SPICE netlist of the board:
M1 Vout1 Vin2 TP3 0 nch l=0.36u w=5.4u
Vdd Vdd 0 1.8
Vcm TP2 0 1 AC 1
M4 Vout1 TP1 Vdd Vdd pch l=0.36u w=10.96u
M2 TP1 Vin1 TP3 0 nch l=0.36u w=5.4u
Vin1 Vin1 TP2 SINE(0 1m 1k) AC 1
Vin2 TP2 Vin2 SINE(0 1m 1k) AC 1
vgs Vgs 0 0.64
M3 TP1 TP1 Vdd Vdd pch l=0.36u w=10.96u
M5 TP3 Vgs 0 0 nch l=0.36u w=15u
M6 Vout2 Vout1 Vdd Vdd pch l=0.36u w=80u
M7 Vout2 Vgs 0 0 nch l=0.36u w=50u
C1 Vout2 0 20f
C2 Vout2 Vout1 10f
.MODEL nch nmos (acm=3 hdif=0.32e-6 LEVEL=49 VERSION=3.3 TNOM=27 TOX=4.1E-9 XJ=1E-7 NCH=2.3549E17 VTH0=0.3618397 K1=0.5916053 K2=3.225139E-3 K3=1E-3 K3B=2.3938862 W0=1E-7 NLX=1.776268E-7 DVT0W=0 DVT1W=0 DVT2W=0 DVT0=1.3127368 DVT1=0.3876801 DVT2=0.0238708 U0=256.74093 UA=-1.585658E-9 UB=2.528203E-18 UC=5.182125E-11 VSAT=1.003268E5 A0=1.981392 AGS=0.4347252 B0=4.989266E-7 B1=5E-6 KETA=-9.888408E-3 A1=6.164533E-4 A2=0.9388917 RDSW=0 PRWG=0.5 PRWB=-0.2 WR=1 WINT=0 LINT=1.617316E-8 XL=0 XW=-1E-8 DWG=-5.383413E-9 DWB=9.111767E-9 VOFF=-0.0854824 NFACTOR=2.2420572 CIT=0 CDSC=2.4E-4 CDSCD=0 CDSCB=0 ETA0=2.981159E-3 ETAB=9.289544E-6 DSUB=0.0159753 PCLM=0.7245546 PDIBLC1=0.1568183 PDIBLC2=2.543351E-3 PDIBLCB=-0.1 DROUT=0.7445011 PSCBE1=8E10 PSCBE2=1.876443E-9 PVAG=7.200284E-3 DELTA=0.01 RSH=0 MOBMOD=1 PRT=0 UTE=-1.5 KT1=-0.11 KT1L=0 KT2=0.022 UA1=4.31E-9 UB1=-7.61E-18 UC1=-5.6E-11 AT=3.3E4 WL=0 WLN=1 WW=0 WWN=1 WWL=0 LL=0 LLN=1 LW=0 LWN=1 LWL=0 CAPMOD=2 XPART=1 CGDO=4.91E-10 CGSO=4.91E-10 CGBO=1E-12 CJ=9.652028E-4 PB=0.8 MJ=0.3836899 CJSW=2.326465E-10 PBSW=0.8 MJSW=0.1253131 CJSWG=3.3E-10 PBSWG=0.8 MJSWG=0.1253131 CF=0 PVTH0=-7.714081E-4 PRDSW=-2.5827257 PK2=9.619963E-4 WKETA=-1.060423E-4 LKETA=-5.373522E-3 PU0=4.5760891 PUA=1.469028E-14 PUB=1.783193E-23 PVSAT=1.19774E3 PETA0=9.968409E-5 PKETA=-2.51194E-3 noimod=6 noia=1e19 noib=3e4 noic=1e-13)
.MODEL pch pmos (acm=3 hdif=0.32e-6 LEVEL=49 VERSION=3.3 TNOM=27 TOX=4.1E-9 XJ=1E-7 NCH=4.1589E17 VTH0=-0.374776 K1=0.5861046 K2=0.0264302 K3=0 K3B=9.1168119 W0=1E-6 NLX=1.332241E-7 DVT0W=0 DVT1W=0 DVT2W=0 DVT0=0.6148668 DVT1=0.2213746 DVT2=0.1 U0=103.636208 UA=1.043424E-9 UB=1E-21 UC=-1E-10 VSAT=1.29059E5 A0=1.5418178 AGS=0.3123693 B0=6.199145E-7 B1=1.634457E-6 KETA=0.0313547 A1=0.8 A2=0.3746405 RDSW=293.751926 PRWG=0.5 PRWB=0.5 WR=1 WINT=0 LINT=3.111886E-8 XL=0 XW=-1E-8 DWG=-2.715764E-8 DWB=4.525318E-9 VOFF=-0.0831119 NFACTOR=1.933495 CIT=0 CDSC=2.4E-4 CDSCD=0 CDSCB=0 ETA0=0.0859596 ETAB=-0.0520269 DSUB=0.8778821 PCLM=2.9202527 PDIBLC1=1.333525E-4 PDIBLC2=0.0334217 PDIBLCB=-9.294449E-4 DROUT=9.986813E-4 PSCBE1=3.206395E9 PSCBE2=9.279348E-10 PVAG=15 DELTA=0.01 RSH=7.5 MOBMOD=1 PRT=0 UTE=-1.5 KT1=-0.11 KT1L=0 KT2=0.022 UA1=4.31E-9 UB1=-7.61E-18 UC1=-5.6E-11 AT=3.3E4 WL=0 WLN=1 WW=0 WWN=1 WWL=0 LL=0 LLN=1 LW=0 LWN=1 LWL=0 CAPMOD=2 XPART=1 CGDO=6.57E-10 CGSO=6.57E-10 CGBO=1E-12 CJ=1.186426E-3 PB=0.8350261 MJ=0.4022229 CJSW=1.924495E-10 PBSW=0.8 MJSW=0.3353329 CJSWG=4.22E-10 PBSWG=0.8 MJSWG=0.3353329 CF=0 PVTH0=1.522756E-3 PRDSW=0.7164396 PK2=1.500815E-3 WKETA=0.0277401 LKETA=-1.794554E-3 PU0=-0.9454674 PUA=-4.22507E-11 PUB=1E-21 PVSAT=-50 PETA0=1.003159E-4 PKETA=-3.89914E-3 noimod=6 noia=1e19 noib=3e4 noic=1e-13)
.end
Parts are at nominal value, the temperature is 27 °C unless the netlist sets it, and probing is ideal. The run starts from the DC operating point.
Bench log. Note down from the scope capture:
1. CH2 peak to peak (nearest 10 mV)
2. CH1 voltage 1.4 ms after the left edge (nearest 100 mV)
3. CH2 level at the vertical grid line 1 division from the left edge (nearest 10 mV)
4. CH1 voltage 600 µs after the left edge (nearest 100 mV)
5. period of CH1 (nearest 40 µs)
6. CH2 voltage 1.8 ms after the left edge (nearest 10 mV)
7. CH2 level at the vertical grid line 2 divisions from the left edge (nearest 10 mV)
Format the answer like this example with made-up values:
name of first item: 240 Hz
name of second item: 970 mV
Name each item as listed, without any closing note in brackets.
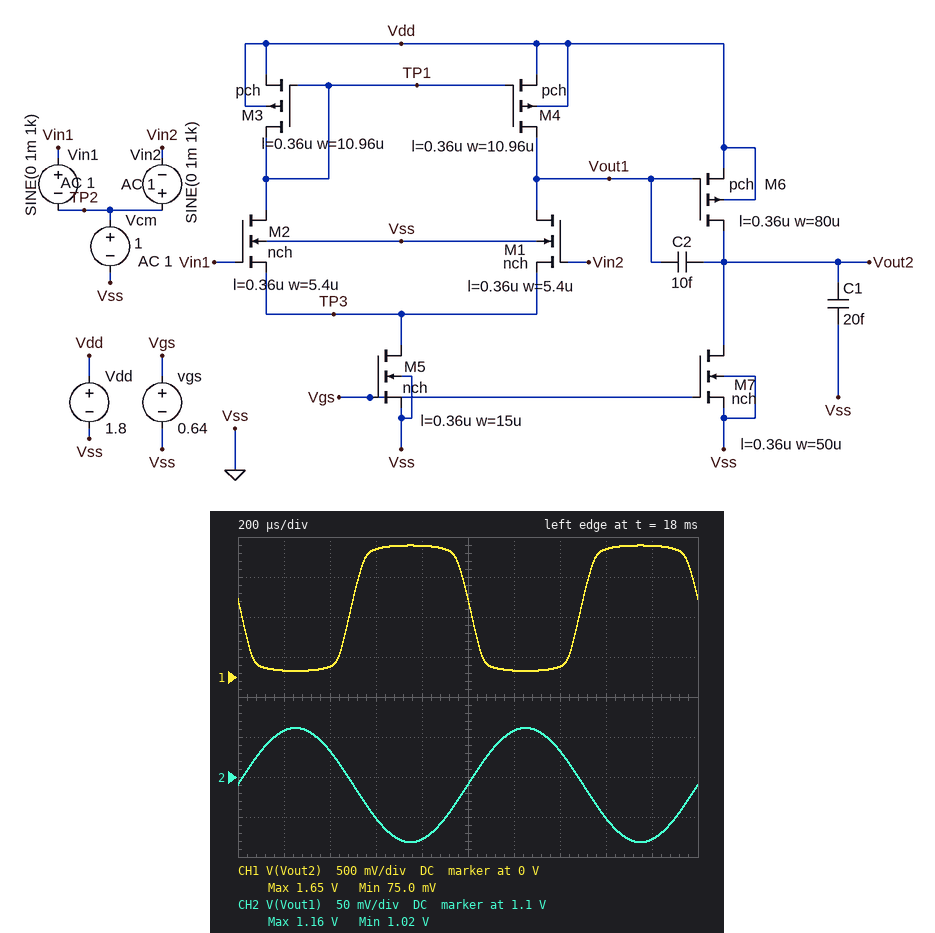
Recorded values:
CH2 peak to peak: 140 mV
CH1 voltage 1.4 ms after the left edge: 100 mV
CH2 level at the vertical grid line 1 division from the left edge: 1.16 V
CH1 voltage 600 µs after the left edge: 1.6 V
period of CH1: 1.00 ms
CH2 voltage 1.8 ms after the left edge: 1.02 V
CH2 level at the vertical grid line 2 divisions from the left edge: 1.13 V
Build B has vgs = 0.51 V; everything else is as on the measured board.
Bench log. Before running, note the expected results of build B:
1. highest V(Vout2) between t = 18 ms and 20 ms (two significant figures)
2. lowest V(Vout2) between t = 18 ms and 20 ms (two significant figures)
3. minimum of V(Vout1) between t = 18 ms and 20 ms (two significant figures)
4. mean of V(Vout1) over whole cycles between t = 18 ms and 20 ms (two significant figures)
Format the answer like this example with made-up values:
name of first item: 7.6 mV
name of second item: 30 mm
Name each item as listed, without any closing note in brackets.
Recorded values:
highest V(Vout2) between t = 18 ms and 20 ms: 1.8 V
lowest V(Vout2) between t = 18 ms and 20 ms: 14 mV
minimum of V(Vout1) between t = 18 ms and 20 ms: 1.2 V
mean of V(Vout1) over whole cycles between t = 18 ms and 20 ms: 1.3 V
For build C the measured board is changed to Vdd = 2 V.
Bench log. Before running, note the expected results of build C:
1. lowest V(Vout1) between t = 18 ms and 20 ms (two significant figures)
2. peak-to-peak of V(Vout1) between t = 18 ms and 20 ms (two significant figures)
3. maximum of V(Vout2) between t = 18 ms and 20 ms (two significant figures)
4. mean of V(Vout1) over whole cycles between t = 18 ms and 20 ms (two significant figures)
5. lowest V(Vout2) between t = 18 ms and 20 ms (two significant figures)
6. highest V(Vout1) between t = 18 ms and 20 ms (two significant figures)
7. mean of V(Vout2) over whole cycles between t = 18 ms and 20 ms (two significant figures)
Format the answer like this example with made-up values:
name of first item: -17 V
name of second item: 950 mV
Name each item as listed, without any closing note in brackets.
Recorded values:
lowest V(Vout1) between t = 18 ms and 20 ms: 1.2 V
peak-to-peak of V(Vout1) between t = 18 ms and 20 ms: 150 mV
maximum of V(Vout2) between t = 18 ms and 20 ms: 1.8 V
mean of V(Vout1) over whole cycles between t = 18 ms and 20 ms: 1.3 V
lowest V(Vout2) between t = 18 ms and 20 ms: 78 mV
highest V(Vout1) between t = 18 ms and 20 ms: 1.4 V
mean of V(Vout2) over whole cycles between t = 18 ms and 20 ms: 980 mV
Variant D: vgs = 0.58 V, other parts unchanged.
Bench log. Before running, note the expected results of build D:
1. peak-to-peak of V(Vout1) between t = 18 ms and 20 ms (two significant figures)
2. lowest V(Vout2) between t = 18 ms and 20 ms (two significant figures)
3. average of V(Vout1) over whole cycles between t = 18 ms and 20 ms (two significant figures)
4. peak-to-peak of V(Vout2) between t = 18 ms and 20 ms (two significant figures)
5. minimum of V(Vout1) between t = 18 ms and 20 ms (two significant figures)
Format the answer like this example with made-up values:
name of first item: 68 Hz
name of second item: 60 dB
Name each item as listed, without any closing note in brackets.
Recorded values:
peak-to-peak of V(Vout1) between t = 18 ms and 20 ms: 160 mV
lowest V(Vout2) between t = 18 ms and 20 ms: 35 mV
average of V(Vout1) over whole cycles between t = 18 ms and 20 ms: 1.2 V
peak-to-peak of V(Vout2) between t = 18 ms and 20 ms: 1.7 V
minimum of V(Vout1) between t = 18 ms and 20 ms: 1.1 V
